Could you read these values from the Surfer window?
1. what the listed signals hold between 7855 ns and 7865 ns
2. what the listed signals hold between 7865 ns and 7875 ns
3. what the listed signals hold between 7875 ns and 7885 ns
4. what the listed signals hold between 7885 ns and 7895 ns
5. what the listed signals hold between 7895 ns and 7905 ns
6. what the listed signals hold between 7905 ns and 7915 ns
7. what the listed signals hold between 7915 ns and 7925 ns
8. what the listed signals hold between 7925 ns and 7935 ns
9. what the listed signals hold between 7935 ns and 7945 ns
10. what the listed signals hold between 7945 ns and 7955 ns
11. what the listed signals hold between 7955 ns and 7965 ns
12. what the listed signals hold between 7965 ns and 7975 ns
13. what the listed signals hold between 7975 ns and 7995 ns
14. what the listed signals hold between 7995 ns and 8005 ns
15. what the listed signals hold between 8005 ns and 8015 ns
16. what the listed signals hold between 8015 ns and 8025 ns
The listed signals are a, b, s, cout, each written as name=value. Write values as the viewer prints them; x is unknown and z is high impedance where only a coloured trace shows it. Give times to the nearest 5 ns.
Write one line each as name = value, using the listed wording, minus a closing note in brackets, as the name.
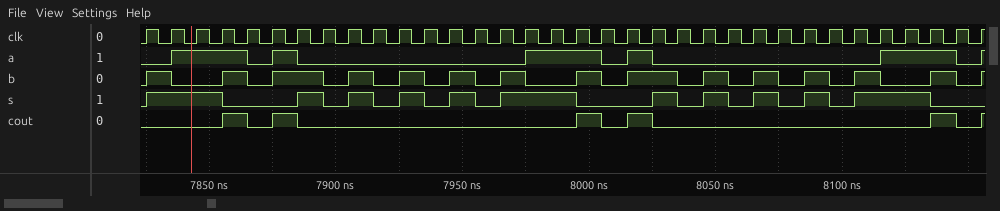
what the listed signals hold between 7855 ns and 7865 ns = a=1, b=1, s=0, cout=1
what the listed signals hold between 7865 ns and 7875 ns = a=0, b=0, s=0, cout=0
what the listed signals hold between 7875 ns and 7885 ns = a=1, b=1, s=0, cout=1
what the listed signals hold between 7885 ns and 7895 ns = a=0, b=1, s=1, cout=0
what the listed signals hold between 7895 ns and 7905 ns = a=0, b=0, s=0, cout=0
what the listed signals hold between 7905 ns and 7915 ns = a=0, b=1, s=1, cout=0
what the listed signals hold between 7915 ns and 7925 ns = a=0, b=0, s=0, cout=0
what the listed signals hold between 7925 ns and 7935 ns = a=0, b=1, s=1, cout=0
what the listed signals hold between 7935 ns and 7945 ns = a=0, b=0, s=0, cout=0
what the listed signals hold between 7945 ns and 7955 ns = a=0, b=1, s=1, cout=0
what the listed signals hold between 7955 ns and 7965 ns = a=0, b=0, s=0, cout=0
what the listed signals hold between 7965 ns and 7975 ns = a=0, b=1, s=1, cout=0
what the listed signals hold between 7975 ns and 7995 ns = a=1, b=0, s=1, cout=0
what the listed signals hold between 7995 ns and 8005 ns = a=1, b=1, s=0, cout=1
what the listed signals hold between 8005 ns and 8015 ns = a=0, b=0, s=0, cout=0
what the listed signals hold between 8015 ns and 8025 ns = a=1, b=1, s=0, cout=1
